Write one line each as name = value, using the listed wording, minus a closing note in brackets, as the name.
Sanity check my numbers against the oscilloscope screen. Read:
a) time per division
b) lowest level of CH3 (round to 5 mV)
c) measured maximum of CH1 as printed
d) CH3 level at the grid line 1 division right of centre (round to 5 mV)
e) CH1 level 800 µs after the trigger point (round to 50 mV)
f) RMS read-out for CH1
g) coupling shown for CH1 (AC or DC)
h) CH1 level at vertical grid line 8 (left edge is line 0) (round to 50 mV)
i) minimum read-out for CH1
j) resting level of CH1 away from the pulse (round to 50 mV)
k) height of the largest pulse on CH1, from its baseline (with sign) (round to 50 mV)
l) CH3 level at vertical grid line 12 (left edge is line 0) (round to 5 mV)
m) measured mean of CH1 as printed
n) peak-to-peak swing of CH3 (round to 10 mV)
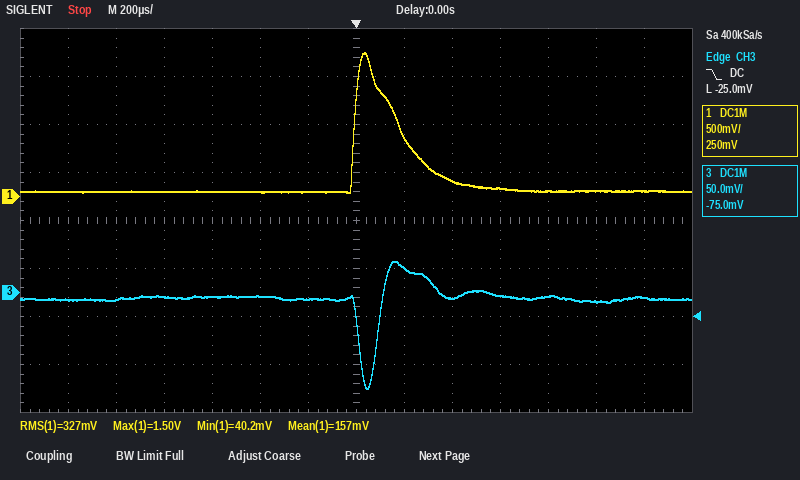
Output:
time per division = 200 µs
lowest level of CH3 = -100 mV
measured maximum of CH1 as printed = 1.50 V
CH3 level at the grid line 1 division right of centre = 25 mV
CH1 level 800 µs after the trigger point = 50 mV
RMS read-out for CH1 = 327 mV
coupling shown for CH1 = DC
CH1 level at vertical grid line 8 (left edge is line 0) = 600 mV
minimum read-out for CH1 = 40.2 mV
resting level of CH1 away from the pulse = 50 mV
height of the largest pulse on CH1, from its baseline (with sign) = +1.45 V
CH3 level at vertical grid line 12 (left edge is line 0) = -10 mV
measured mean of CH1 as printed = 157 mV
peak-to-peak swing of CH3 = 130 mV
